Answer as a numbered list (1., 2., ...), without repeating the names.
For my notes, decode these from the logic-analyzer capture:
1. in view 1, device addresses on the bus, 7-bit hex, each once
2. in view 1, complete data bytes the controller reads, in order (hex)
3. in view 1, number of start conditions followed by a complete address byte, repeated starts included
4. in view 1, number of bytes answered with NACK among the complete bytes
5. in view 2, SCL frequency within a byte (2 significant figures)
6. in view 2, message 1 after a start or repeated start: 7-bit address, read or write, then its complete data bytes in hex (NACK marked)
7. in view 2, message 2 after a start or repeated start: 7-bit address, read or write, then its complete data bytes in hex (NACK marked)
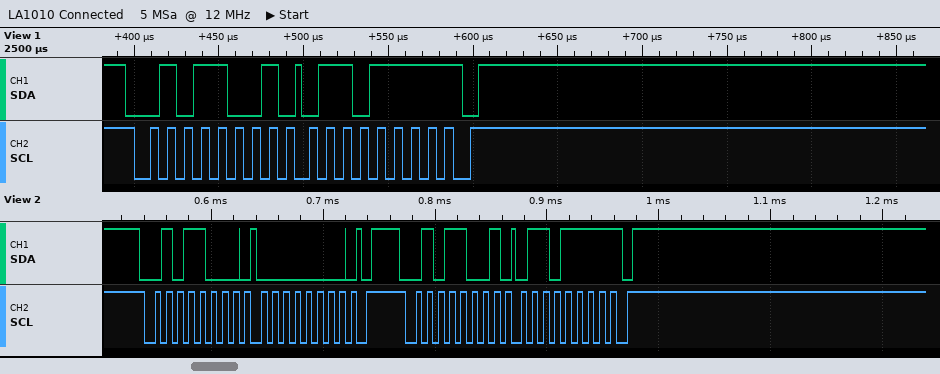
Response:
1. 0x2C
2. 6F
3. 1
4. 1
5. 100 kHz
6. 0x2C write: 00
7. 0x2C read: 6F NACK
